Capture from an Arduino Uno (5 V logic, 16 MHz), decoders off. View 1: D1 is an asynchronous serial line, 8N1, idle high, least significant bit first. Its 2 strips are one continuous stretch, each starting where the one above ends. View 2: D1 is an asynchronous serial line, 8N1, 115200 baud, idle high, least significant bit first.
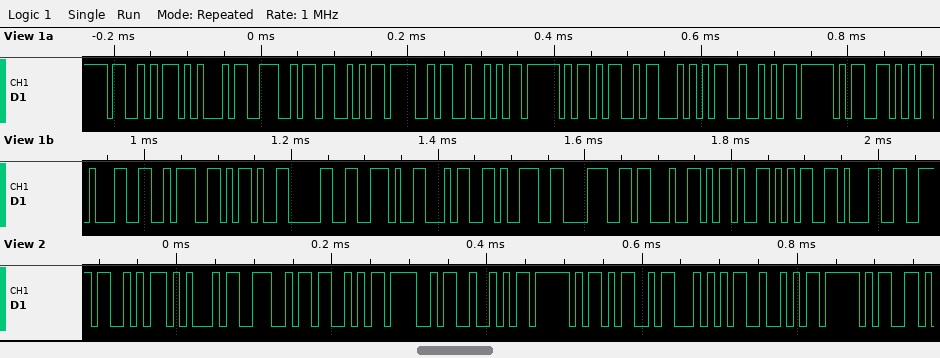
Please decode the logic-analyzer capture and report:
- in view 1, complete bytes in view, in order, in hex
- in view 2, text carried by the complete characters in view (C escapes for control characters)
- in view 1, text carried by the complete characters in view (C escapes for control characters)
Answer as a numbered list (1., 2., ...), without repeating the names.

1. 53 45 4E 53 4F 52 5F 4D 54 52 5F 56 31 3A 2D 30 2E 34 39 38 23 2D 35 31
2. "SENSOR_MTR_"
3. "SENSOR_MTR_V1:-0.498#-51"
